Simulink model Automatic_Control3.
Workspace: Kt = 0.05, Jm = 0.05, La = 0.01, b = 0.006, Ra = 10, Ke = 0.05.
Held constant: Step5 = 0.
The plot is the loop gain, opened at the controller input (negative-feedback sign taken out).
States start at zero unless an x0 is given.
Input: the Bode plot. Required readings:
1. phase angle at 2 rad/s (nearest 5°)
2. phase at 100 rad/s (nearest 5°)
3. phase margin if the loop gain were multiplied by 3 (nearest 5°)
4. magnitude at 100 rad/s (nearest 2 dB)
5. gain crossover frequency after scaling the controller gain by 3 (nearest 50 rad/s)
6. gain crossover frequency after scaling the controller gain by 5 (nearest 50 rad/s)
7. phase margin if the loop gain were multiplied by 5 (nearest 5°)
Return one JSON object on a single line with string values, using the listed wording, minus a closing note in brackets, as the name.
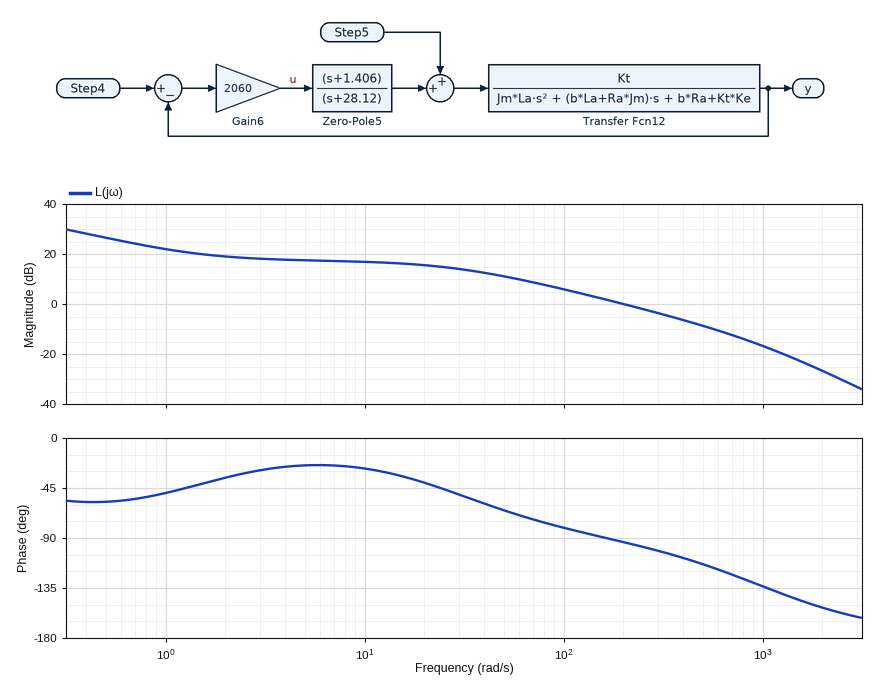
{"phase angle at 2 rad/s": "-35°", "phase at 100 rad/s": "-80°", "phase margin if the loop gain were multiplied by 3": "65°", "magnitude at 100 rad/s": "6 dB", "gain crossover frequency after scaling the controller gain by 3": "550 rad/s", "gain crossover frequency after scaling the controller gain by 5": "800 rad/s", "phase margin if the loop gain were multiplied by 5": "55°"}
